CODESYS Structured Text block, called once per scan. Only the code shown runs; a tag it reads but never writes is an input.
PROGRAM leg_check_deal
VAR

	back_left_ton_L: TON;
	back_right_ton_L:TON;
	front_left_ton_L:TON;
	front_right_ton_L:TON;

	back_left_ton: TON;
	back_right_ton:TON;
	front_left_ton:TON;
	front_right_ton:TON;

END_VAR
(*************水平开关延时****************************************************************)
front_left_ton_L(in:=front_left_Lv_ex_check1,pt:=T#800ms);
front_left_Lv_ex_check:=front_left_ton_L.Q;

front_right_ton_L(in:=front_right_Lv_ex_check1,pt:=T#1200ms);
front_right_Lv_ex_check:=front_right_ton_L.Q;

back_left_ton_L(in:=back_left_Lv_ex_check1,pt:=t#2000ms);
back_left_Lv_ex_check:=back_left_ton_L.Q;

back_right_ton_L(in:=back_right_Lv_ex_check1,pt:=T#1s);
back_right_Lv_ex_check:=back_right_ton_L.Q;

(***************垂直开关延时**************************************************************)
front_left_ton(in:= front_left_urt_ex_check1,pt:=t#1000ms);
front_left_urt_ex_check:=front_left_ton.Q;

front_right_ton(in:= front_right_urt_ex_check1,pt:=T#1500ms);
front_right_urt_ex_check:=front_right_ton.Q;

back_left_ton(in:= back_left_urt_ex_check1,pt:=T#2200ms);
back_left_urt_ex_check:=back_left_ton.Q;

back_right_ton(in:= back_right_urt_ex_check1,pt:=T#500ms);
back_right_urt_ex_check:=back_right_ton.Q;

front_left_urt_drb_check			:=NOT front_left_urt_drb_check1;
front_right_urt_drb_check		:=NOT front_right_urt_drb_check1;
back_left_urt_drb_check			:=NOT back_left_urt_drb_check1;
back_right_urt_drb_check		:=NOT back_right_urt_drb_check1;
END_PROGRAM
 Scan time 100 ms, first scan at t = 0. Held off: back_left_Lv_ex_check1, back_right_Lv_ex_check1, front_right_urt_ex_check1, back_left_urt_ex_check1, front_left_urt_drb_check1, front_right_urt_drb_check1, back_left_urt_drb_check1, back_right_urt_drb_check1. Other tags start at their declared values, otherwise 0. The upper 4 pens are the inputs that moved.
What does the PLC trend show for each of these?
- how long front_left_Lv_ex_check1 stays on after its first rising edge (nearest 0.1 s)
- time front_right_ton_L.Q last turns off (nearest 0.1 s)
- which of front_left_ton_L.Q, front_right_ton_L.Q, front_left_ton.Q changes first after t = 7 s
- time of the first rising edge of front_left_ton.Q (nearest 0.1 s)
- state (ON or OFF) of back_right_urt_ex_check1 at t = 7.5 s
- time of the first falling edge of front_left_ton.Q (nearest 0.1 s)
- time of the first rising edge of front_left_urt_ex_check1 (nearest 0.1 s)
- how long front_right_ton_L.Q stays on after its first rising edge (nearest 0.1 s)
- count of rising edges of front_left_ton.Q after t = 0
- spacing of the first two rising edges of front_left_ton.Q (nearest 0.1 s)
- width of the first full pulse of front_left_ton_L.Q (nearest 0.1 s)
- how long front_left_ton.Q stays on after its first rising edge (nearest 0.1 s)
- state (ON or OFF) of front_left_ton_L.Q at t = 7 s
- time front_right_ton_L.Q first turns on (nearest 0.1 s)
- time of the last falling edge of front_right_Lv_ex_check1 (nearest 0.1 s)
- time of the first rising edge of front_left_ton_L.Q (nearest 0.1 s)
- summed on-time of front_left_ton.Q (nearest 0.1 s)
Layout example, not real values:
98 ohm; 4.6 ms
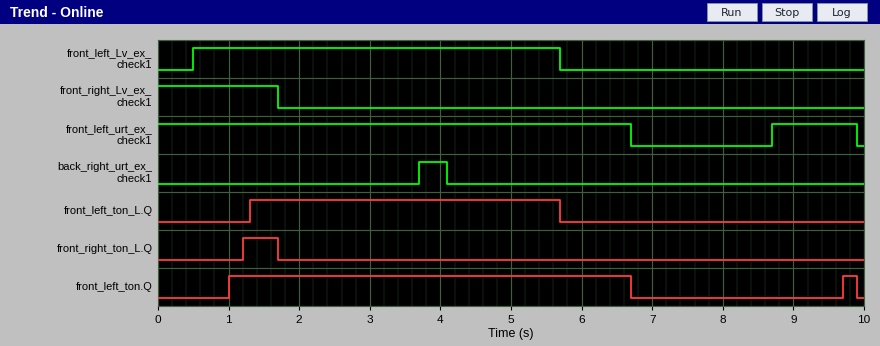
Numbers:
5.2 s; 1.7 s; front_left_ton.Q; 1.0 s; OFF; 6.7 s; 8.7 s; 0.5 s; 2; 8.7 s; 4.4 s; 5.7 s; OFF; 1.2 s; 1.7 s; 1.3 s; 5.9 s
